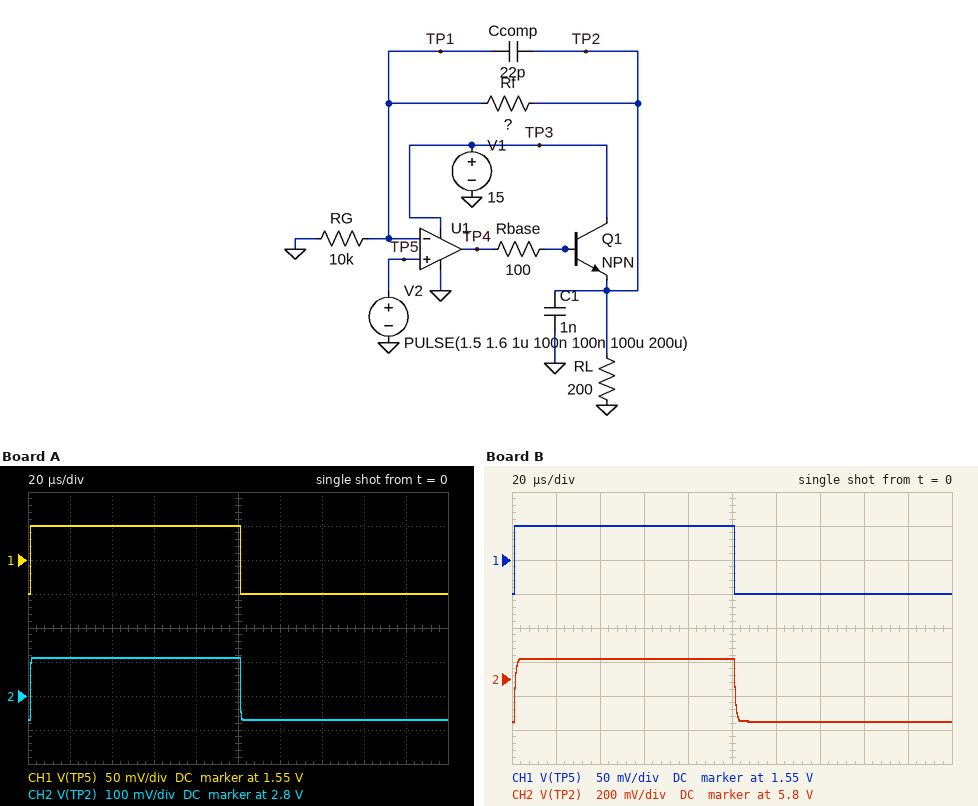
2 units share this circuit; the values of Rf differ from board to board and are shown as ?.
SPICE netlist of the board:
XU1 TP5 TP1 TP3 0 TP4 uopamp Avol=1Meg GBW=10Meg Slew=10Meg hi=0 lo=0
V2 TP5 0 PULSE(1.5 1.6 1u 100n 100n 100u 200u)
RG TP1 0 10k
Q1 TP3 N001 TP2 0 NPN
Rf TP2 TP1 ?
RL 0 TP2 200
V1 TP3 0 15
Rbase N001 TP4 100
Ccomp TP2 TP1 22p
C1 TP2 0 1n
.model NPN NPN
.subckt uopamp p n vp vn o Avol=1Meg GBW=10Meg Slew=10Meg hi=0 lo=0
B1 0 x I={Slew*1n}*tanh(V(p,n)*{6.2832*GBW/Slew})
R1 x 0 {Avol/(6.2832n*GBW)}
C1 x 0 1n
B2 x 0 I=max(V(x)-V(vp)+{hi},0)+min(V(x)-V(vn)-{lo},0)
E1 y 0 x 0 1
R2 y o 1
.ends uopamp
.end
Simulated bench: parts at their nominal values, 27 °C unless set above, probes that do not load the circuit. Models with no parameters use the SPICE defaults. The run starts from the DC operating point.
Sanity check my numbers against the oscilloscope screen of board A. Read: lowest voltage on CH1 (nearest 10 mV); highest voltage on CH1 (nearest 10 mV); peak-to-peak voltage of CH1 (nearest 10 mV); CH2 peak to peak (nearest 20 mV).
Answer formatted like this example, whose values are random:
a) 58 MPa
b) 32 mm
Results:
a) 1.50 V
b) 1.60 V
c) 100 mV
d) 180 mV
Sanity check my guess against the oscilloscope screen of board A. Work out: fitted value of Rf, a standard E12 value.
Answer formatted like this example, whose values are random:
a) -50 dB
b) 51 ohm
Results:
a) 8.2 kΩ
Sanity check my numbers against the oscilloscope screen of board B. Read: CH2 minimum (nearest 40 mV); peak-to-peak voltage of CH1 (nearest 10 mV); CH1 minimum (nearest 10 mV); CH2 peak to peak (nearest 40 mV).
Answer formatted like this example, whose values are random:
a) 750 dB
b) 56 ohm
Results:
a) 5.56 V
b) 100 mV
c) 1.50 V
d) 360 mV
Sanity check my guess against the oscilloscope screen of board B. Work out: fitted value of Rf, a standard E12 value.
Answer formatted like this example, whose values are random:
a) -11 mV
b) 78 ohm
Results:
a) 27 kΩ
